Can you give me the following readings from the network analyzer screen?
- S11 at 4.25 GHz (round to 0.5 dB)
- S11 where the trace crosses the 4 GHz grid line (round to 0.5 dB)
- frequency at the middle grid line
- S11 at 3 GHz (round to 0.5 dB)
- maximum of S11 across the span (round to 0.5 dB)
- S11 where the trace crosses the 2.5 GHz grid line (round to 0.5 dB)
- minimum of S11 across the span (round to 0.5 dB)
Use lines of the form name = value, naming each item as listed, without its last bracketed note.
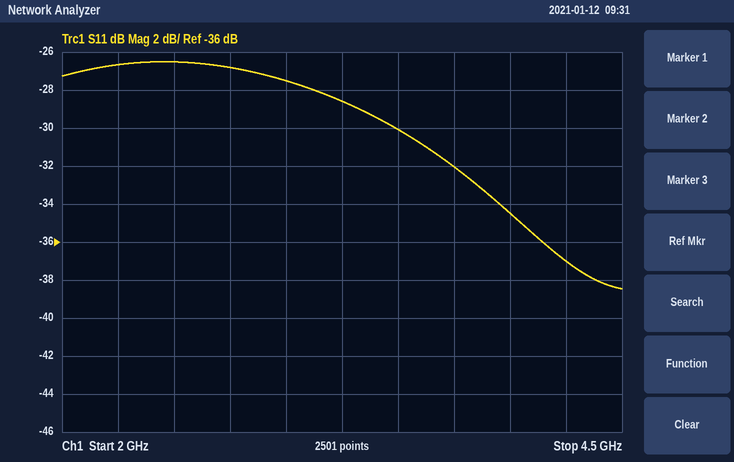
S11 at 4.25 GHz = -37.0 dB
S11 where the trace crosses the 4 GHz grid line = -34.5 dB
frequency at the middle grid line = 3.25 GHz
S11 at 3 GHz = -27.5 dB
maximum of S11 across the span = -26.5 dB
S11 where the trace crosses the 2.5 GHz grid line = -26.5 dB
minimum of S11 across the span = -38.5 dB
